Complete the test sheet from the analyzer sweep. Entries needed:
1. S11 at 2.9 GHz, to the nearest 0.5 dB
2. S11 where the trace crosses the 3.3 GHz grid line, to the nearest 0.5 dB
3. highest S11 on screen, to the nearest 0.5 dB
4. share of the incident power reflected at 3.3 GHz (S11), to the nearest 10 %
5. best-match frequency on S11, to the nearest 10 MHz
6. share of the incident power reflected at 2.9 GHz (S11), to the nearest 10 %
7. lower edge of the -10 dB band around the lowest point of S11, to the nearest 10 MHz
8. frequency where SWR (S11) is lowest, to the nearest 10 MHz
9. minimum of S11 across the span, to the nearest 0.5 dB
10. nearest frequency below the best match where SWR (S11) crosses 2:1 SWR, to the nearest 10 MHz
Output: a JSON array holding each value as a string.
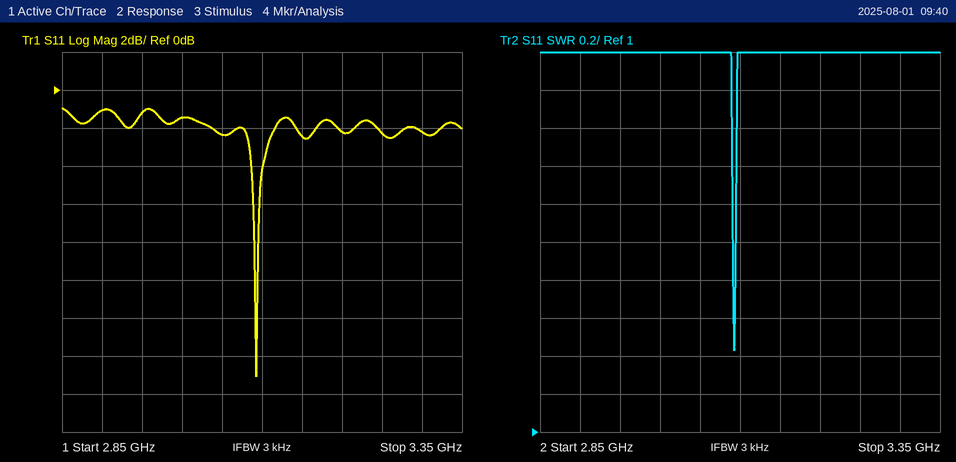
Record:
["-1.0 dB", "-2.0 dB", "-1.0 dB", "60 %", "3.09 GHz", "80 %", "3.09 GHz", "3.09 GHz", "-15.0 dB", "3.09 GHz"]
